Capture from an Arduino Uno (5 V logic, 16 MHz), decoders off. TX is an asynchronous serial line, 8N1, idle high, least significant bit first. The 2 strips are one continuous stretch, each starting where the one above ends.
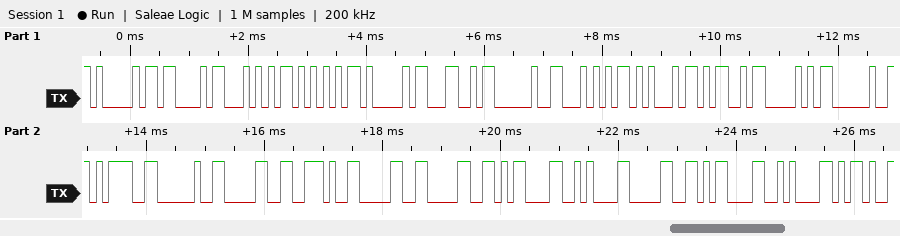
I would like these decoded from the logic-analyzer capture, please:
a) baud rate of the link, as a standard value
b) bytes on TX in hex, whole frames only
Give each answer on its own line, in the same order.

9600 baud
41 43 54 55 41 4C 20 54 45 4D 50 20 3D 20 30 2E 30 30 0D 0A 30 0D 0A 2D
